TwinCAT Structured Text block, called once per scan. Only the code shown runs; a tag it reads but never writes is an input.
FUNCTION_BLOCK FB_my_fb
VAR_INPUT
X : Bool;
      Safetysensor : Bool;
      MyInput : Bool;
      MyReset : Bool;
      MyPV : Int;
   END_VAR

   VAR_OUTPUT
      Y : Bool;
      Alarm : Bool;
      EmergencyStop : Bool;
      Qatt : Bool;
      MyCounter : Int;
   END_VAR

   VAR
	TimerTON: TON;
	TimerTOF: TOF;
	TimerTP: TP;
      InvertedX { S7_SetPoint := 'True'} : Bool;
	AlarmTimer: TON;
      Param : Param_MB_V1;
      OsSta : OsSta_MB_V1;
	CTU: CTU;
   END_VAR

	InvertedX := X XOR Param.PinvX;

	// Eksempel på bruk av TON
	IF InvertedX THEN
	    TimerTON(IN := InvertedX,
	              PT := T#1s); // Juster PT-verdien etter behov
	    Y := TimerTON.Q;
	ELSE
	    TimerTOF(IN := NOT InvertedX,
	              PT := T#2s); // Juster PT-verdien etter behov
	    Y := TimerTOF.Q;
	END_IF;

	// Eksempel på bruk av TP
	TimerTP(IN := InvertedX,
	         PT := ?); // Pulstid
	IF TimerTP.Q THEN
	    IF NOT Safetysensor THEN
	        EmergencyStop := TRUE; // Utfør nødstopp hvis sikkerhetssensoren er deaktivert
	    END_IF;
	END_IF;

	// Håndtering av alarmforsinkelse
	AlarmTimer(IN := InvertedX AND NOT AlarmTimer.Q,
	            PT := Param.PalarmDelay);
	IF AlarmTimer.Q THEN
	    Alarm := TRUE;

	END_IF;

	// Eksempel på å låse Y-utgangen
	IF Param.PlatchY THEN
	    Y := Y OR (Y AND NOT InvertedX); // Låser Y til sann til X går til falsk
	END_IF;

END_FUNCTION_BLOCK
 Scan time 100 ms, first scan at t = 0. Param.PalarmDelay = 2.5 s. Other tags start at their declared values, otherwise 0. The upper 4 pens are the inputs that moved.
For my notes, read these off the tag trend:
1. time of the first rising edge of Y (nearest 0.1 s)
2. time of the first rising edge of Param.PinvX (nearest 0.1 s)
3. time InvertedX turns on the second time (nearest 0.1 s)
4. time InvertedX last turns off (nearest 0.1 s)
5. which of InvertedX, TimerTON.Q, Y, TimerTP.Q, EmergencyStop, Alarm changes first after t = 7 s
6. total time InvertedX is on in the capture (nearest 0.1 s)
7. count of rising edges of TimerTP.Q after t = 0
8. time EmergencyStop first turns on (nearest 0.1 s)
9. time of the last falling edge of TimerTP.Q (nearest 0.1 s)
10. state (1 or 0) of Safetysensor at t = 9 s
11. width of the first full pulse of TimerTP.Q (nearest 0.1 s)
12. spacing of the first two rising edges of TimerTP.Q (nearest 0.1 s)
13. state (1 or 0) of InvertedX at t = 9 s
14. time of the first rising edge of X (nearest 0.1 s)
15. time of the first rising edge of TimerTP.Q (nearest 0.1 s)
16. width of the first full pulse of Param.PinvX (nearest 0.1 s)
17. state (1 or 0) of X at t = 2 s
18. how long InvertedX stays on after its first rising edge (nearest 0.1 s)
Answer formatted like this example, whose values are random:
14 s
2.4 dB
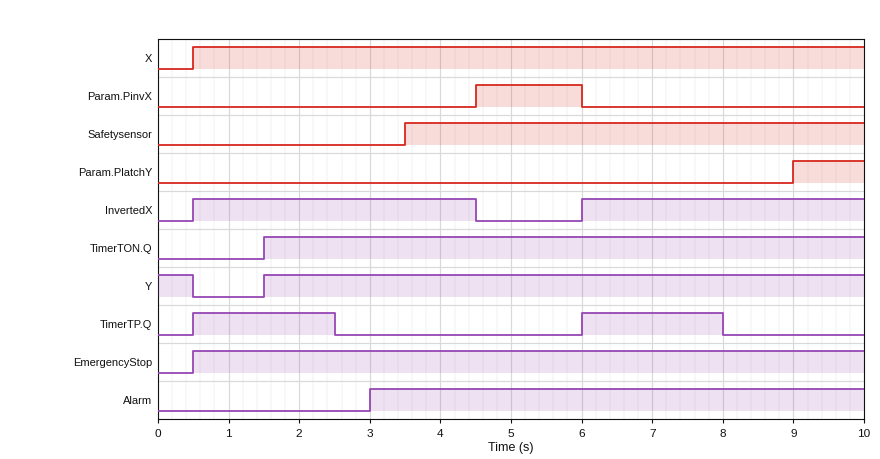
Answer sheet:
1.5 s
4.5 s
6.0 s
4.5 s
TimerTP.Q
8.0 s
2
0.5 s
8.0 s
1
2.0 s
5.5 s
1
0.5 s
0.5 s
1.5 s
1
4.0 s
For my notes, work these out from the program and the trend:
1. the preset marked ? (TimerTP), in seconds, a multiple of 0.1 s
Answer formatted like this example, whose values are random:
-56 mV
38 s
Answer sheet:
2.0 s
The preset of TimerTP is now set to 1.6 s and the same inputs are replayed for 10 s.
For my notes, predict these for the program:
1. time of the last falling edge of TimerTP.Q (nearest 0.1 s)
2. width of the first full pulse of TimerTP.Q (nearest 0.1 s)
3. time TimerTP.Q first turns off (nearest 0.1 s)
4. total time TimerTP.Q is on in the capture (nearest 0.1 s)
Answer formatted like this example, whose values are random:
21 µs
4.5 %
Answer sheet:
7.6 s
1.6 s
2.1 s
3.2 s
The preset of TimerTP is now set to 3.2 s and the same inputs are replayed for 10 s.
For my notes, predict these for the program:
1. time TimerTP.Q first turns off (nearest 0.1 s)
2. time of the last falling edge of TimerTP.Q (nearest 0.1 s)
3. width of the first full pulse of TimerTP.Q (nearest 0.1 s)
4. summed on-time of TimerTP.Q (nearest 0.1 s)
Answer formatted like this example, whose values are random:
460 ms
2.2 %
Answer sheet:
3.7 s
9.2 s
3.2 s
6.4 s
